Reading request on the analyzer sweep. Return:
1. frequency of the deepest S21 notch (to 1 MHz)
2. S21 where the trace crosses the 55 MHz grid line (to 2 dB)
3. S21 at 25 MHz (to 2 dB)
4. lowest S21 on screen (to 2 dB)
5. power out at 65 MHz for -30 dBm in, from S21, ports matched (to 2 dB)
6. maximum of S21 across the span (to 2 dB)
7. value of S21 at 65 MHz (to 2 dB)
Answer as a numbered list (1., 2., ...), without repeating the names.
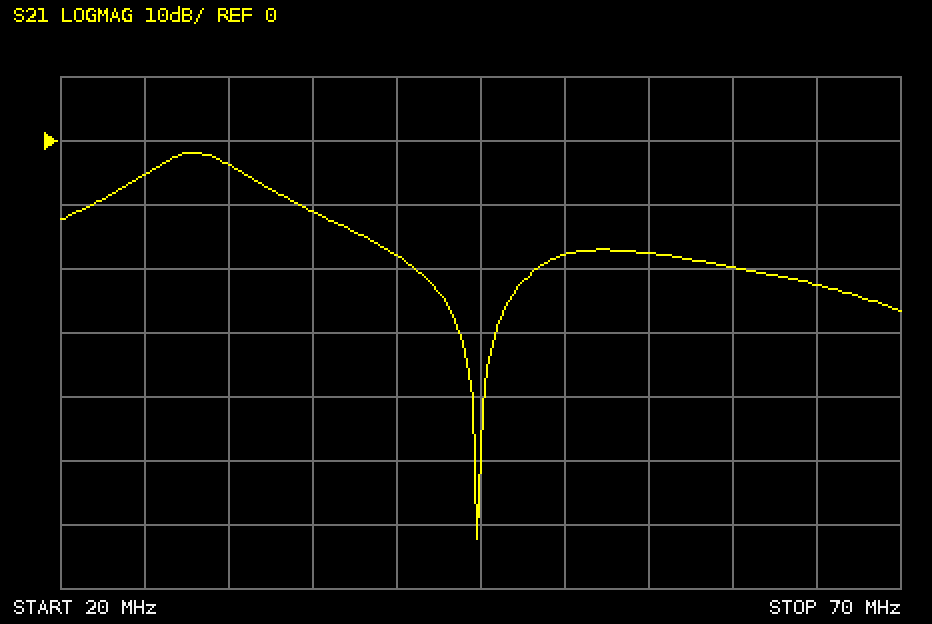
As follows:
1. 45 MHz
2. -18 dB
3. -6 dB
4. -62 dB
5. -52 dBm
6. -2 dB
7. -22 dB
